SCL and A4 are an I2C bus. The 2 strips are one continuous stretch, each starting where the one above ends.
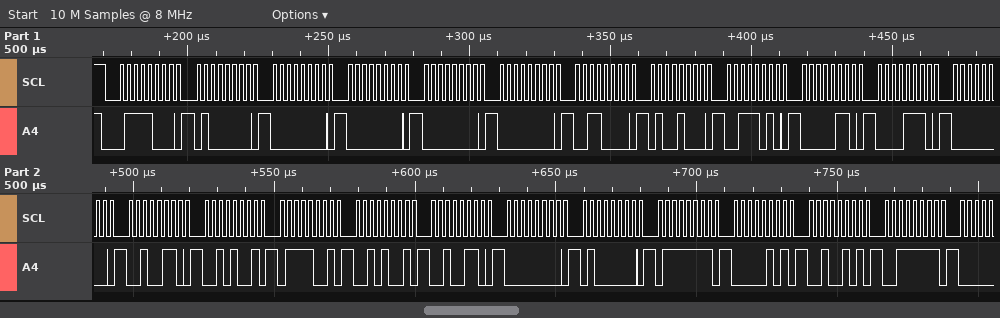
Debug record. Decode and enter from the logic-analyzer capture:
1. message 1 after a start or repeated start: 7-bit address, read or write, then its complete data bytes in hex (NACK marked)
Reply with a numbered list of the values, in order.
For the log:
1. 0x3C write: 40 00 00 00 00 30 48 3A 06 0E 00 26 29 79 29 26 00 40 7F 05 25 3F
